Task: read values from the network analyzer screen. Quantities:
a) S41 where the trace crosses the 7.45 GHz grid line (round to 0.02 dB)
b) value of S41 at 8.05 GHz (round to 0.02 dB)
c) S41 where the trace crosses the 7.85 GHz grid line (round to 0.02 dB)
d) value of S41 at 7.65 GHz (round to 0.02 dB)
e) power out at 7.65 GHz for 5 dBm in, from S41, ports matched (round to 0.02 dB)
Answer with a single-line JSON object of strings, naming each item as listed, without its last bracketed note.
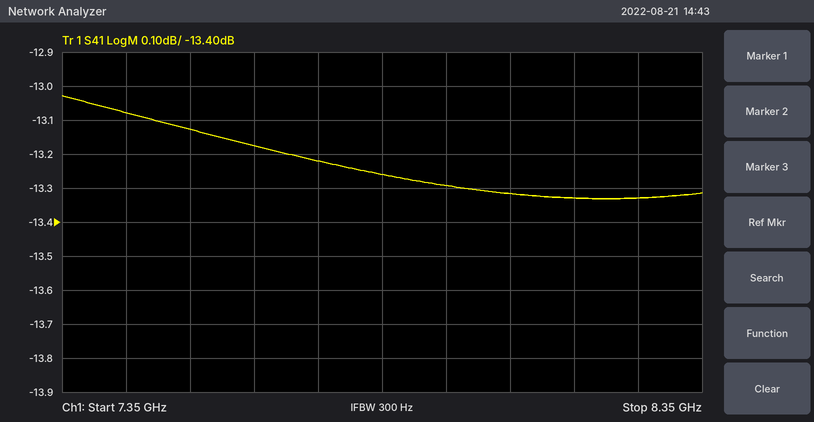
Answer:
{"S41 where the trace crosses the 7.45 GHz grid line": "-13.08 dB", "value of S41 at 8.05 GHz": "-13.32 dB", "S41 where the trace crosses the 7.85 GHz grid line": "-13.26 dB", "value of S41 at 7.65 GHz": "-13.18 dB", "power out at 7.65 GHz for 5 dBm in, from S41, ports matched": "-8.18 dBm"}
